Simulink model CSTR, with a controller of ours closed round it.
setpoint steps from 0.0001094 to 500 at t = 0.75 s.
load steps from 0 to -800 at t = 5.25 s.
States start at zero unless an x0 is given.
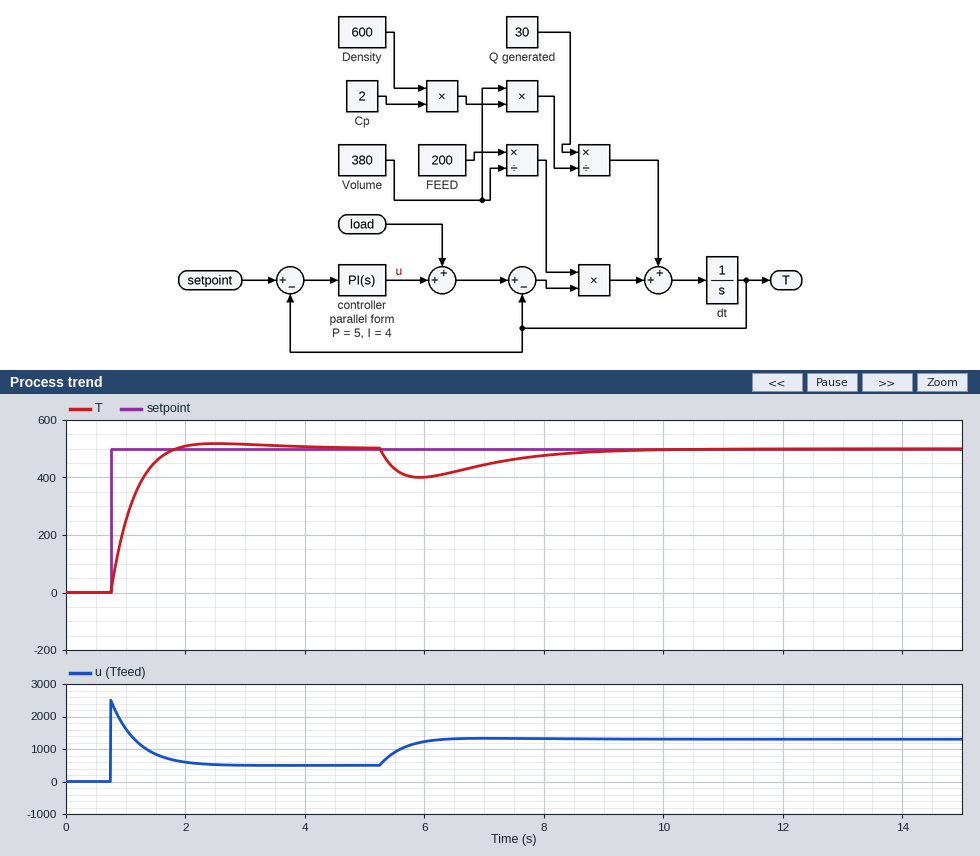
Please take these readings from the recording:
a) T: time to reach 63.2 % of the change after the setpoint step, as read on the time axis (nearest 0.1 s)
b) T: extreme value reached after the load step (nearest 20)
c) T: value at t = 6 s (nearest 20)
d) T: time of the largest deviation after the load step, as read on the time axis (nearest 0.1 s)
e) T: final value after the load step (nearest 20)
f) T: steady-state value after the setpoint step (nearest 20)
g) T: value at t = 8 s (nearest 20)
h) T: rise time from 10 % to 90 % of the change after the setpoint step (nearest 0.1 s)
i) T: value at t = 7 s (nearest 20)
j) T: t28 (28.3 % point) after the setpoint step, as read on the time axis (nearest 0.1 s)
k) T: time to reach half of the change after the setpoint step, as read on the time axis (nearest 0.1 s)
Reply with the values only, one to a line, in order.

1.1 s
400
400
5.9 s
500
500
480
0.7 s
440
0.9 s
1.0 s
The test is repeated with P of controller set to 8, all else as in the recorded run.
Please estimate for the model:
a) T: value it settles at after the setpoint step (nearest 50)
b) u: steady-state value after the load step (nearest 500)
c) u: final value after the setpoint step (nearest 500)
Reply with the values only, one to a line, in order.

500
1500
500
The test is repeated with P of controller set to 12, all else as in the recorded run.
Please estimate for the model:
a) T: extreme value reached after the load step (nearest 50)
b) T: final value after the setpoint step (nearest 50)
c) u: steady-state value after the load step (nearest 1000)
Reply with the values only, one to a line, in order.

450
500
1000
